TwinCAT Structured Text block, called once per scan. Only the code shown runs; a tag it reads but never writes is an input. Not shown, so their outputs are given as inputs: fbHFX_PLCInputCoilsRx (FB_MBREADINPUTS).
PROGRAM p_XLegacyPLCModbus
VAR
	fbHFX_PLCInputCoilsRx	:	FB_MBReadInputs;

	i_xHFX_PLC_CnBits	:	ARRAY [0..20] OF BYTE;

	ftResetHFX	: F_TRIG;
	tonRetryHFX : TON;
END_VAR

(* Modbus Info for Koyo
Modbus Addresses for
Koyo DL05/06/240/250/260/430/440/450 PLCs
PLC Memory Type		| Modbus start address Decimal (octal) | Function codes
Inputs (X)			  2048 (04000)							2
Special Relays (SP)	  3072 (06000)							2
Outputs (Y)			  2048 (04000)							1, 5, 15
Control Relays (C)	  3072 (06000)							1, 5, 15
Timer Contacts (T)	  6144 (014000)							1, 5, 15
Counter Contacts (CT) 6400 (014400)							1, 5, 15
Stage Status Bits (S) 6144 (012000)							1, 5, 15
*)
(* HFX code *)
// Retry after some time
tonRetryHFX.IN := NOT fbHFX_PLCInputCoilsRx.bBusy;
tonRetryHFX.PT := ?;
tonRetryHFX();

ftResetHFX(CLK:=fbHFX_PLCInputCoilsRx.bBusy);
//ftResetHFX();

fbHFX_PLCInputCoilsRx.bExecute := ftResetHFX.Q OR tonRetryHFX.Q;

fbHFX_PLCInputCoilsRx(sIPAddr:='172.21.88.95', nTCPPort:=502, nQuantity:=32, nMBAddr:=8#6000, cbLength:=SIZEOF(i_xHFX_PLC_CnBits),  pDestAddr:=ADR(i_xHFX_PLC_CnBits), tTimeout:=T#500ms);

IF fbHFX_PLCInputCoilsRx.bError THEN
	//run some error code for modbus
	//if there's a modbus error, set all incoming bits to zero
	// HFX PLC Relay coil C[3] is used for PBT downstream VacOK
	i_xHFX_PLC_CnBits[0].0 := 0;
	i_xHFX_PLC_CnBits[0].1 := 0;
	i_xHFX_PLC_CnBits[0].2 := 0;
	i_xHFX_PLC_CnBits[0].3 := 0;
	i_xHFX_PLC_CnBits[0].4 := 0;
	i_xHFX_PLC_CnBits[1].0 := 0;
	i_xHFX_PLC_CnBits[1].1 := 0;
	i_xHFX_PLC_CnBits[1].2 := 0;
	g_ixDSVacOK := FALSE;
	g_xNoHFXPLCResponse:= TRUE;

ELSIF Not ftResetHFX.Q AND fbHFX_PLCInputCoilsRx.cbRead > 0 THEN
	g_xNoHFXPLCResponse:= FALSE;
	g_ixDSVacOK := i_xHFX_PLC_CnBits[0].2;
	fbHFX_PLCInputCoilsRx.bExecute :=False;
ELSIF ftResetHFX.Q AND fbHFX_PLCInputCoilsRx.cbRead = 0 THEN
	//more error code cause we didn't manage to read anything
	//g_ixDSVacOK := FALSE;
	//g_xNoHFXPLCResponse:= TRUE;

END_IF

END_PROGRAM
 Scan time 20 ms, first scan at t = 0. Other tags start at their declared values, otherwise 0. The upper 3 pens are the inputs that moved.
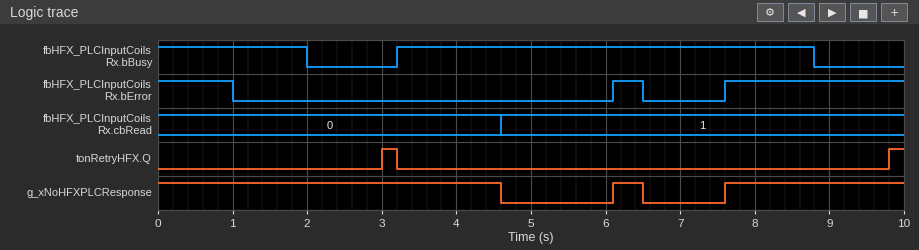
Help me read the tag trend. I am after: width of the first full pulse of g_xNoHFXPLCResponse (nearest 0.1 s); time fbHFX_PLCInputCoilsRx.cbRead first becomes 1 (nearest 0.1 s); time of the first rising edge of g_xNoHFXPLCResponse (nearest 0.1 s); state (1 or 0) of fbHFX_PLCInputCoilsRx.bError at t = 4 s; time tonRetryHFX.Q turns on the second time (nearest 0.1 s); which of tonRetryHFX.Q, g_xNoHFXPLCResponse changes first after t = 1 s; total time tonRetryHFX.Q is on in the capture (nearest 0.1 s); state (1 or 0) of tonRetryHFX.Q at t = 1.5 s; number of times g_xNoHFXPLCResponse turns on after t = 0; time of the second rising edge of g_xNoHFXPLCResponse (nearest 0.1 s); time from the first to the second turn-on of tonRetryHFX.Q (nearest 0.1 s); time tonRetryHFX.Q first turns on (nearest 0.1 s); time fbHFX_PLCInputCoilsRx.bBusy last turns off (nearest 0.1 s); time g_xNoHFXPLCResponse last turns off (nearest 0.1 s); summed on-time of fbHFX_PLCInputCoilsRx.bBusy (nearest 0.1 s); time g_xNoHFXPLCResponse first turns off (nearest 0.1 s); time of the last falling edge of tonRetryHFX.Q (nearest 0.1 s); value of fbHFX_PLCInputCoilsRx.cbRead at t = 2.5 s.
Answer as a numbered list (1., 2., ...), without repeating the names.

1. 0.4 s
2. 4.6 s
3. 6.1 s
4. 0
5. 9.8 s
6. tonRetryHFX.Q
7. 0.4 s
8. 0
9. 2
10. 7.6 s
11. 6.8 s
12. 3.0 s
13. 8.8 s
14. 6.5 s
15. 7.6 s
16. 4.6 s
17. 3.2 s
18. 0
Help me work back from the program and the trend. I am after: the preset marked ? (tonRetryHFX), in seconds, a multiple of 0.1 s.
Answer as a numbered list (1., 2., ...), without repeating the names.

1. 1.0 s
